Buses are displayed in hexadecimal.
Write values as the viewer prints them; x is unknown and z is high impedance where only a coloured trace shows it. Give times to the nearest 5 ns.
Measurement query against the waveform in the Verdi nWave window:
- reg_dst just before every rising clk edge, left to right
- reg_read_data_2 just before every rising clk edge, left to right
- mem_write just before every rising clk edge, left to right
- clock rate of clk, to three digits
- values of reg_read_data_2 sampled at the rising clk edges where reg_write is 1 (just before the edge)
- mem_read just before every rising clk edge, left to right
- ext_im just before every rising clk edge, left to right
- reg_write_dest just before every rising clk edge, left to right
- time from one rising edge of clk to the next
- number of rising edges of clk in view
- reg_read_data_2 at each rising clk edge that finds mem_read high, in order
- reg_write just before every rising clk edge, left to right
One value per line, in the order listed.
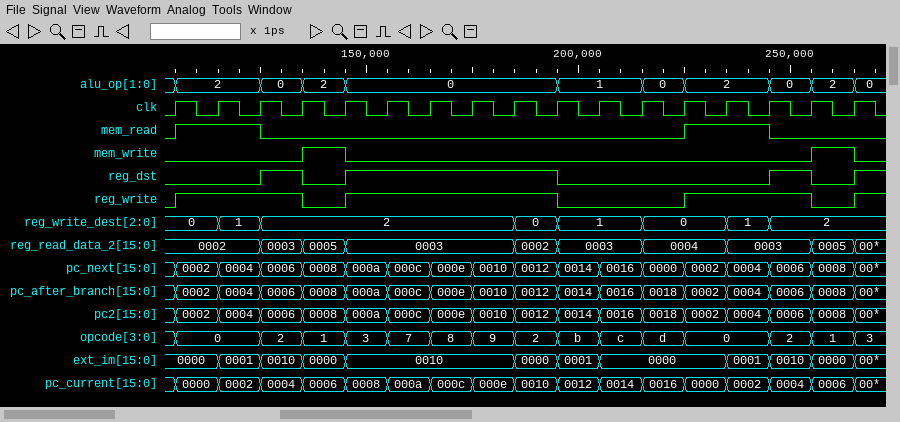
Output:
0 0 0 1 0 1 1 1 1 1 0 0 0 0 0 1 0
0002, 0002, 0002, 0003, 0005, 0003, 0003, 0003, 0003, 0002, 0003, 0003, 0004, 0004, 0003, 0003, 0005
0 0 0 0 1 0 0 0 0 0 0 0 0 0 0 0 1
100 MHz
0002, 0002, 0003, 0003, 0003, 0003, 0003, 0002, 0004, 0003, 0003
0 1 1 0 0 0 0 0 0 0 0 0 0 1 1 0 0
0000, 0000, 0001, 0010, 0000, 0010, 0010, 0010, 0010, 0000, 0001, 0000, 0000, 0000, 0001, 0010, 0000
0, 0, 1, 2, 2, 2, 2, 2, 2, 0, 1, 1, 0, 0, 1, 2, 2
10 ns
17
0002, 0002, 0004, 0003
0 1 1 1 0 1 1 1 1 1 0 0 0 1 1 1 0
